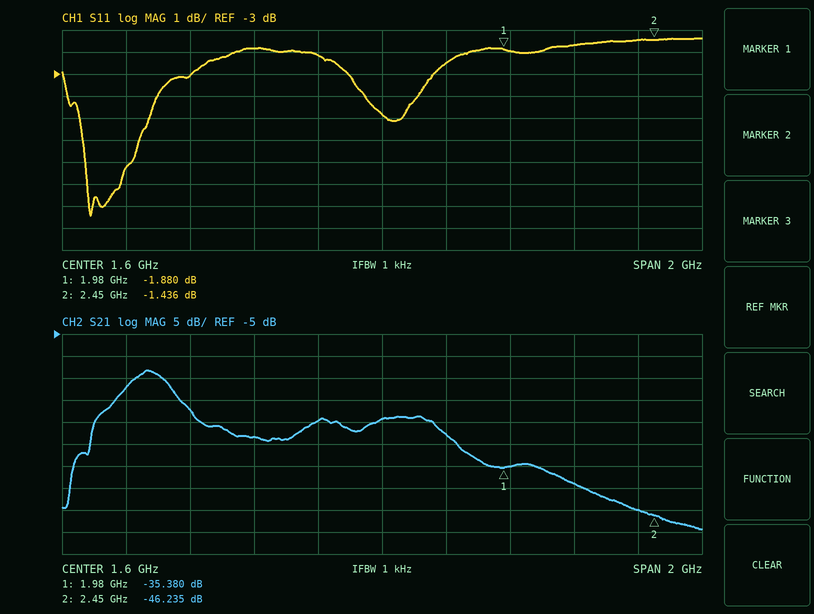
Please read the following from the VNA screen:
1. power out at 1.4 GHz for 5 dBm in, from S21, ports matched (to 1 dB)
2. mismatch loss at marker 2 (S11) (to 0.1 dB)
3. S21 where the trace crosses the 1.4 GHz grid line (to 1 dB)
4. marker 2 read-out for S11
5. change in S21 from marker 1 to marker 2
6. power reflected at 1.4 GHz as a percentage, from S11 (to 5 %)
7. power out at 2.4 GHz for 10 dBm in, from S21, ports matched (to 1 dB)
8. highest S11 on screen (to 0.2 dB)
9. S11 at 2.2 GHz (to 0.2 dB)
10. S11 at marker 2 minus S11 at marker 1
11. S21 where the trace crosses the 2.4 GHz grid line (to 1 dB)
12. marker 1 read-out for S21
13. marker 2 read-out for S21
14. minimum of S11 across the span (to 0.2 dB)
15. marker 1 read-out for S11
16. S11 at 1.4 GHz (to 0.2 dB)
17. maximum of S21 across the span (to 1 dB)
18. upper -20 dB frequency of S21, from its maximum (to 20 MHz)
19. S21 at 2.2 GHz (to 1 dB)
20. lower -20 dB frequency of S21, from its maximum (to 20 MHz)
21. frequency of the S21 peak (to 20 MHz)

-20 dBm
5.5 dB
-25 dB
-1.436 dB
-10.855 dB
60 %
-35 dBm
-1.4 dB
-1.6 dB
0.444 dB
-45 dB
-35.380 dB
-46.235 dB
-9.4 dB
-1.880 dB
-2.2 dB
-13 dB
1.90 GHz
-39 dB
640 MHz
860 MHz
